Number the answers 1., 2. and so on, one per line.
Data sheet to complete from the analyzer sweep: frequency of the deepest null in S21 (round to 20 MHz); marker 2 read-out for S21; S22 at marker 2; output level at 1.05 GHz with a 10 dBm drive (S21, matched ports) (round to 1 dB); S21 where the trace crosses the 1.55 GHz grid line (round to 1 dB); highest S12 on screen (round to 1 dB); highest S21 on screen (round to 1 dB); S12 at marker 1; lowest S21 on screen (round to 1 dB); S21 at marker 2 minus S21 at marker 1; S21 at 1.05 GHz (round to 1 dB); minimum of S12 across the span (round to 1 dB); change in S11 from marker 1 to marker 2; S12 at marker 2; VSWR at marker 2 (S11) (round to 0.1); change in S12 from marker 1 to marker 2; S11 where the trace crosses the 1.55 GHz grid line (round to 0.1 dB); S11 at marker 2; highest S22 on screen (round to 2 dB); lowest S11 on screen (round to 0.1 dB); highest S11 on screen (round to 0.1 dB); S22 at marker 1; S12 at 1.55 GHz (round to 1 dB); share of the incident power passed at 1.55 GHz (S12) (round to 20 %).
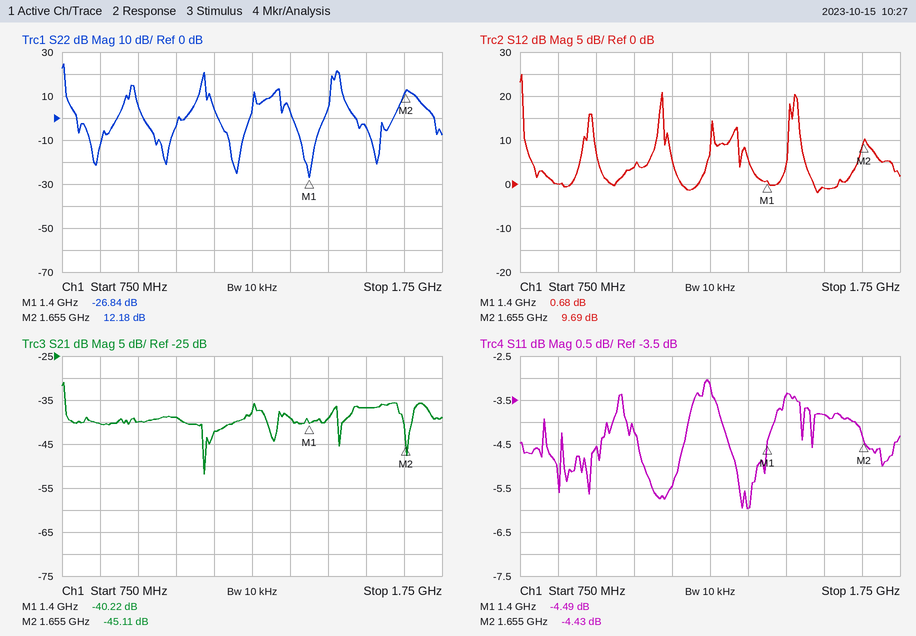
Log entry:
1. 1.12 GHz
2. -45.11 dB
3. 12.18 dB
4. -29 dBm
5. -37 dB
6. 25 dB
7. -31 dB
8. 0.68 dB
9. -52 dB
10. -4.89 dB
11. -39 dB
12. -2 dB
13. 0.06 dB
14. 9.69 dB
15. 4.0
16. 9.01 dB
17. -3.8 dB
18. -4.43 dB
19. 24 dB
20. -6.0 dB
21. -3.0 dB
22. -26.84 dB
23. -1 dB
24. 80 %
